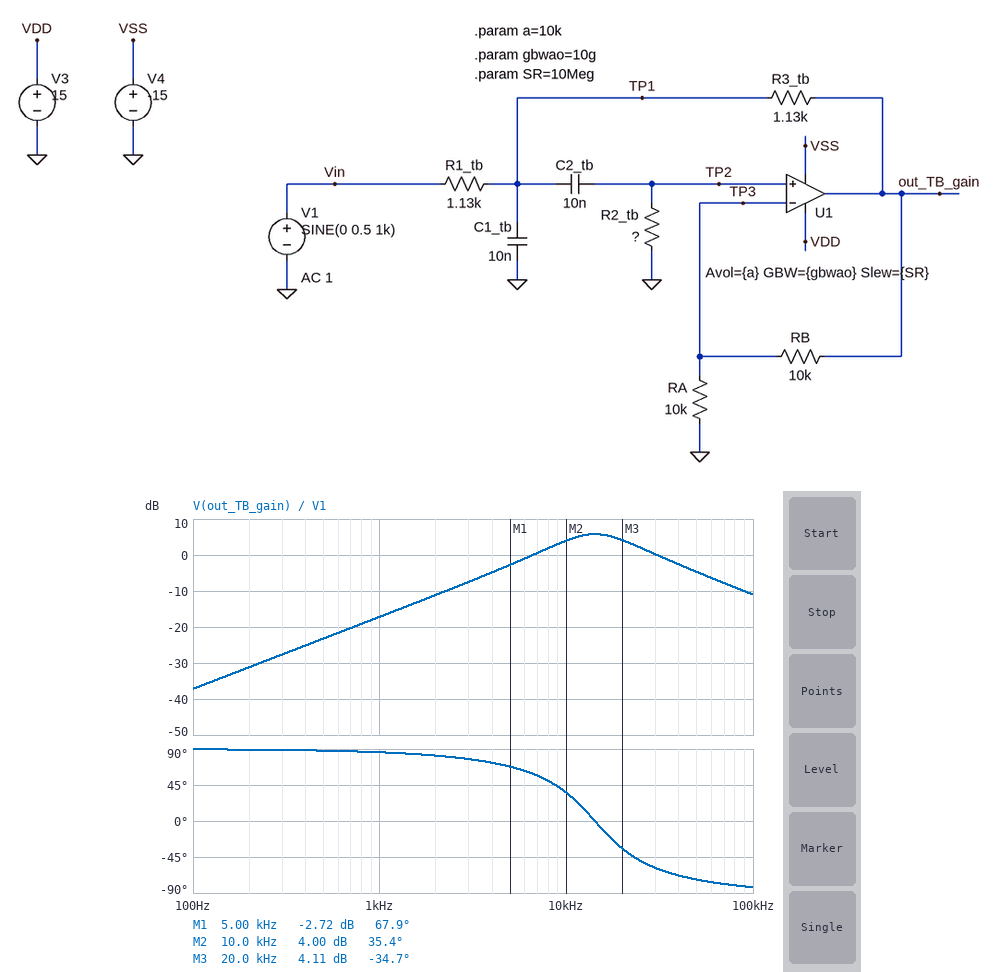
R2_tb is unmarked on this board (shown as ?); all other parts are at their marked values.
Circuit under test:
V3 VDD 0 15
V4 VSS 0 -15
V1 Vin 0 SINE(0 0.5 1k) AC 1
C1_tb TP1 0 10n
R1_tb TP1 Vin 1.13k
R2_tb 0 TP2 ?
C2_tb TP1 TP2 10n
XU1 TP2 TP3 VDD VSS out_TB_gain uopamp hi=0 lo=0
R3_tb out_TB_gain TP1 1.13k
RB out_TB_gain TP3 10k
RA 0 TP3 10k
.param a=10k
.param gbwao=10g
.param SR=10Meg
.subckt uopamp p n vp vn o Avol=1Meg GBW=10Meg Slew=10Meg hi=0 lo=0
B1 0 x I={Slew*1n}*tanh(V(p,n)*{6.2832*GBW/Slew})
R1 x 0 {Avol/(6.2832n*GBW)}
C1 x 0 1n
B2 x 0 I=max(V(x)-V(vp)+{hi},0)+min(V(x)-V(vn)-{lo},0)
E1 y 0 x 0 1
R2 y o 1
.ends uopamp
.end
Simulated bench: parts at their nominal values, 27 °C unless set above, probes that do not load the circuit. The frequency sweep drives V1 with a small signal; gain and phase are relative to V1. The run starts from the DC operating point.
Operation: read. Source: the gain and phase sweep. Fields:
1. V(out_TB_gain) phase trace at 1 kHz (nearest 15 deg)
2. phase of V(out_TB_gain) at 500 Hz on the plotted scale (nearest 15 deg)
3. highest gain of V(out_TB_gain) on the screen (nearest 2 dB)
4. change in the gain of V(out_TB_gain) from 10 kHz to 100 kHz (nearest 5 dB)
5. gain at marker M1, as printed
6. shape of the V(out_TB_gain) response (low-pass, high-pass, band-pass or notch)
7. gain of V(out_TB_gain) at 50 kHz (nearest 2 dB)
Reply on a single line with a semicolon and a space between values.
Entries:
90 deg; 90 deg; 6 dB; -15 dB; -2.72 dB; band-pass; -4 dB
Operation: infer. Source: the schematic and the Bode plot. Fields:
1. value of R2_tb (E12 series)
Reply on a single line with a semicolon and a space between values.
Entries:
2.2 kΩ
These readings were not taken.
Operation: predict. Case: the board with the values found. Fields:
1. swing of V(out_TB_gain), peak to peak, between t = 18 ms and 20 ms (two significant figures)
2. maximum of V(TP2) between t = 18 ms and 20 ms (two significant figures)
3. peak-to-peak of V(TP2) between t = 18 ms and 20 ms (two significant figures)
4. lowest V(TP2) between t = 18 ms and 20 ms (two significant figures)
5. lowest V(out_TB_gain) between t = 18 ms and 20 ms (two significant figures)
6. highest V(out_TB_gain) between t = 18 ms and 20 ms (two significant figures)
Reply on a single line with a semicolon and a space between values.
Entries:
140 mV; 35 mV; 69 mV; -35 mV; -69 mV; 69 mV
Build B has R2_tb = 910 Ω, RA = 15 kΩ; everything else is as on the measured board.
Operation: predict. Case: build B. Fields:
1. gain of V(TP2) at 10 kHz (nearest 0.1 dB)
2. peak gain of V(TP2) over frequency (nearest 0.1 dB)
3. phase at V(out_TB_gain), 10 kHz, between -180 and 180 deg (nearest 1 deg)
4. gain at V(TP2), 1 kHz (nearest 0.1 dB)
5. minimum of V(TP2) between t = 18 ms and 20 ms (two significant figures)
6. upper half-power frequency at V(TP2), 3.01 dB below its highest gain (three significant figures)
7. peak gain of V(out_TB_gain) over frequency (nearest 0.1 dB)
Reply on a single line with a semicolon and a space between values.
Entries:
-12.0 dB; -9.0 dB; 45 deg; -30.9 dB; -14 mV; 49.4 kHz; -4.6 dB
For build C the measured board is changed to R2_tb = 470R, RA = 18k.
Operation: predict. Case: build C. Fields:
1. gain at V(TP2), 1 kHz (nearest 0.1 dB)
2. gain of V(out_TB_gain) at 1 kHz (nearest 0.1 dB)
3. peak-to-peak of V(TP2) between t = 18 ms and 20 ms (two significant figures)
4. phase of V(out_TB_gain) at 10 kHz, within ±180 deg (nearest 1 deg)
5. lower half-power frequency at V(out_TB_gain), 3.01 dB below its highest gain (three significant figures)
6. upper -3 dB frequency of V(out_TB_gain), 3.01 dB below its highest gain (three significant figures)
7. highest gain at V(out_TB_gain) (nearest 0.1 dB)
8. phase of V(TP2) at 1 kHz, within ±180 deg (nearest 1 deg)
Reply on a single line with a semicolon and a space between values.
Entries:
-36.6 dB; -32.8 dB; 15 mV; 49 deg; 11.2 kHz; 84.9 kHz; -10.6 dB; 86 deg
